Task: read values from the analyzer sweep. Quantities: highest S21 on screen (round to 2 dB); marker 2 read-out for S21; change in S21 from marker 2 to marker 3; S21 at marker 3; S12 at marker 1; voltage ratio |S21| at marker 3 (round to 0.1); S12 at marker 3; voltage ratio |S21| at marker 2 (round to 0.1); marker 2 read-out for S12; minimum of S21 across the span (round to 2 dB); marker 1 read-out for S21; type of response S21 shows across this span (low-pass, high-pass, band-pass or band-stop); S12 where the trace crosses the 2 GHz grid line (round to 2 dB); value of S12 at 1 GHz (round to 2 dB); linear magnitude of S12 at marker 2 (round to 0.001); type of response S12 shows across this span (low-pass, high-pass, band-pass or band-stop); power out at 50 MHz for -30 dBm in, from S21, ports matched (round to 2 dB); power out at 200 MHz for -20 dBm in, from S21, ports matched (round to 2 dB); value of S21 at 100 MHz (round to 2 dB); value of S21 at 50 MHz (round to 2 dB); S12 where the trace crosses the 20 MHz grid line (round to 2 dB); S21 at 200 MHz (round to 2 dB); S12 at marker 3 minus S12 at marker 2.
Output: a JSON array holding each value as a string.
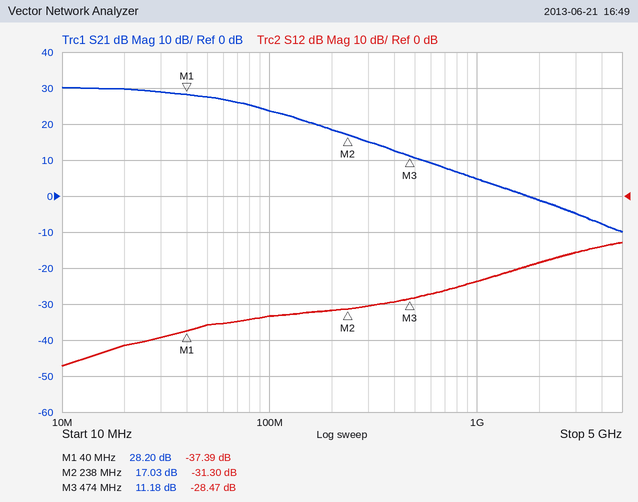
["30 dB", "17.03 dB", "-5.85 dB", "11.18 dB", "-37.39 dB", "3.6", "-28.47 dB", "7.1", "-31.30 dB", "-10 dB", "28.20 dB", "low-pass", "-18 dB", "-24 dB", "0.027", "high-pass", "-2 dBm", "-2 dBm", "24 dB", "28 dB", "-42 dB", "18 dB", "2.83 dB"]
